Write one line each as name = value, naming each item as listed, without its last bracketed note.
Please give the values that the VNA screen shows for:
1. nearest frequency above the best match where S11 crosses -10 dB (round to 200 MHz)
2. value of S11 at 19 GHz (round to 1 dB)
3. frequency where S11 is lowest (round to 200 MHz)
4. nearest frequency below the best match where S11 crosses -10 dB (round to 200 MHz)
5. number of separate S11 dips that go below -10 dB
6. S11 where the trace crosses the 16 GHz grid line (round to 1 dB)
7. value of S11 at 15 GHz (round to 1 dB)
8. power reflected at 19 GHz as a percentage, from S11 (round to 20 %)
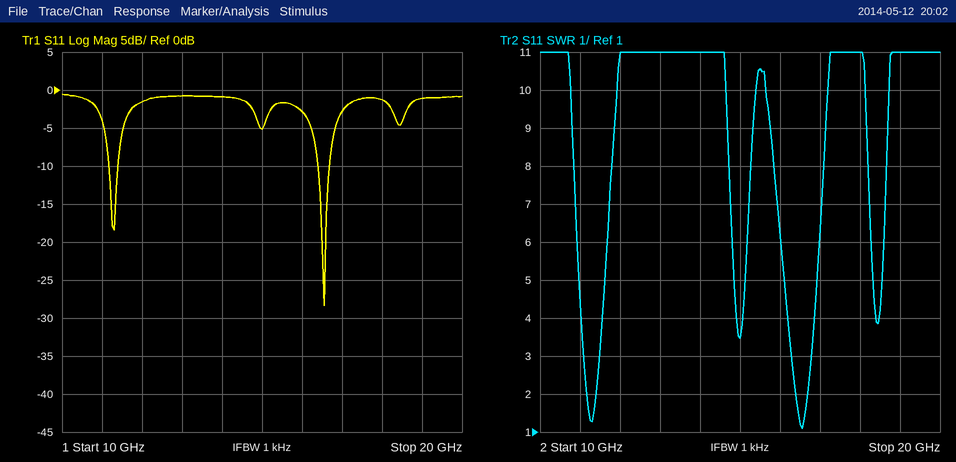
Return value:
nearest frequency above the best match where S11 crosses -10 dB = 16.6 GHz
value of S11 at 19 GHz = -1 dB
frequency where S11 is lowest = 16.6 GHz
nearest frequency below the best match where S11 crosses -10 dB = 16.4 GHz
number of separate S11 dips that go below -10 dB = 2
S11 where the trace crosses the 16 GHz grid line = -3 dB
value of S11 at 15 GHz = -5 dB
power reflected at 19 GHz as a percentage, from S11 = 80 %
